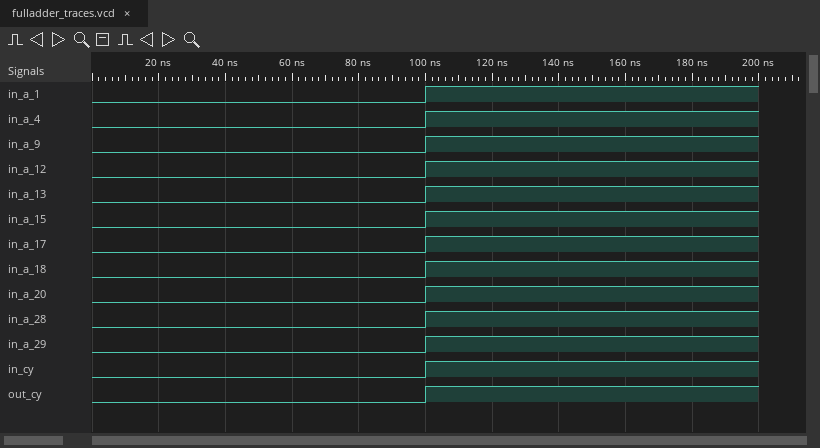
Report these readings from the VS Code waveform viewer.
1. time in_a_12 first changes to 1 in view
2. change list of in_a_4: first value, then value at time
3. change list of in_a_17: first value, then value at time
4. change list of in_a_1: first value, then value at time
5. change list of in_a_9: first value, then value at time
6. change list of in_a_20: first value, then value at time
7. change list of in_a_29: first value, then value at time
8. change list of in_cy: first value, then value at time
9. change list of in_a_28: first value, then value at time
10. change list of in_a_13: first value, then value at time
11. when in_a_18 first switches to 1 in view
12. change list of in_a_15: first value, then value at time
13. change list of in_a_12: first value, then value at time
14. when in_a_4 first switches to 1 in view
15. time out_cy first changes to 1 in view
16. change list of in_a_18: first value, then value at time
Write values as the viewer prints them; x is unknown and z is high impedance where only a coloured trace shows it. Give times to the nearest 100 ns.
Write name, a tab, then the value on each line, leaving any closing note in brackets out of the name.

time in_a_12 first changes to 1 in view	100 ns
change list of in_a_4: first value, then value at time	0, 1 at 100 ns
change list of in_a_17: first value, then value at time	0, 1 at 100 ns
change list of in_a_1: first value, then value at time	0, 1 at 100 ns
change list of in_a_9: first value, then value at time	0, 1 at 100 ns
change list of in_a_20: first value, then value at time	0, 1 at 100 ns
change list of in_a_29: first value, then value at time	0, 1 at 100 ns
change list of in_cy: first value, then value at time	0, 1 at 100 ns
change list of in_a_28: first value, then value at time	0, 1 at 100 ns
change list of in_a_13: first value, then value at time	0, 1 at 100 ns
when in_a_18 first switches to 1 in view	100 ns
change list of in_a_15: first value, then value at time	0, 1 at 100 ns
change list of in_a_12: first value, then value at time	0, 1 at 100 ns
when in_a_4 first switches to 1 in view	100 ns
time out_cy first changes to 1 in view	100 ns
change list of in_a_18: first value, then value at time	0, 1 at 100 ns
